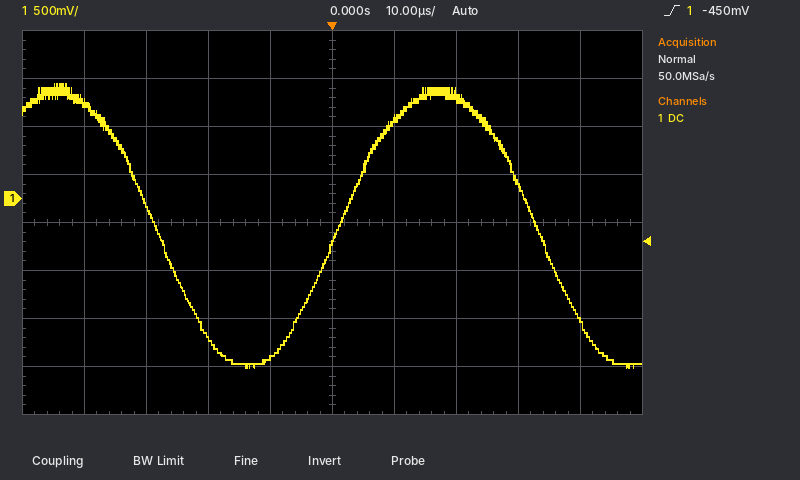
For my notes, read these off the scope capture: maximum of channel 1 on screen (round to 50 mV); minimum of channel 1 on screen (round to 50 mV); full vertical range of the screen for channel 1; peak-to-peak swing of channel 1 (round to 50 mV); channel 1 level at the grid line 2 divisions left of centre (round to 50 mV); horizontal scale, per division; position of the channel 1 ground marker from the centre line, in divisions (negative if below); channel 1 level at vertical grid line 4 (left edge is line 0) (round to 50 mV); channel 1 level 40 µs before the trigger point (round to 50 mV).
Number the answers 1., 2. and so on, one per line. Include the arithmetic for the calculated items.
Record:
1. 1.20 V
2. -1.75 V
3. 4 V
4. 1.20 V − (-1.75 V) = 2.95 V
5. -1.45 V
6. 10 µs
7. +0.5 div
8. -1.65 V
9. 1.00 V
